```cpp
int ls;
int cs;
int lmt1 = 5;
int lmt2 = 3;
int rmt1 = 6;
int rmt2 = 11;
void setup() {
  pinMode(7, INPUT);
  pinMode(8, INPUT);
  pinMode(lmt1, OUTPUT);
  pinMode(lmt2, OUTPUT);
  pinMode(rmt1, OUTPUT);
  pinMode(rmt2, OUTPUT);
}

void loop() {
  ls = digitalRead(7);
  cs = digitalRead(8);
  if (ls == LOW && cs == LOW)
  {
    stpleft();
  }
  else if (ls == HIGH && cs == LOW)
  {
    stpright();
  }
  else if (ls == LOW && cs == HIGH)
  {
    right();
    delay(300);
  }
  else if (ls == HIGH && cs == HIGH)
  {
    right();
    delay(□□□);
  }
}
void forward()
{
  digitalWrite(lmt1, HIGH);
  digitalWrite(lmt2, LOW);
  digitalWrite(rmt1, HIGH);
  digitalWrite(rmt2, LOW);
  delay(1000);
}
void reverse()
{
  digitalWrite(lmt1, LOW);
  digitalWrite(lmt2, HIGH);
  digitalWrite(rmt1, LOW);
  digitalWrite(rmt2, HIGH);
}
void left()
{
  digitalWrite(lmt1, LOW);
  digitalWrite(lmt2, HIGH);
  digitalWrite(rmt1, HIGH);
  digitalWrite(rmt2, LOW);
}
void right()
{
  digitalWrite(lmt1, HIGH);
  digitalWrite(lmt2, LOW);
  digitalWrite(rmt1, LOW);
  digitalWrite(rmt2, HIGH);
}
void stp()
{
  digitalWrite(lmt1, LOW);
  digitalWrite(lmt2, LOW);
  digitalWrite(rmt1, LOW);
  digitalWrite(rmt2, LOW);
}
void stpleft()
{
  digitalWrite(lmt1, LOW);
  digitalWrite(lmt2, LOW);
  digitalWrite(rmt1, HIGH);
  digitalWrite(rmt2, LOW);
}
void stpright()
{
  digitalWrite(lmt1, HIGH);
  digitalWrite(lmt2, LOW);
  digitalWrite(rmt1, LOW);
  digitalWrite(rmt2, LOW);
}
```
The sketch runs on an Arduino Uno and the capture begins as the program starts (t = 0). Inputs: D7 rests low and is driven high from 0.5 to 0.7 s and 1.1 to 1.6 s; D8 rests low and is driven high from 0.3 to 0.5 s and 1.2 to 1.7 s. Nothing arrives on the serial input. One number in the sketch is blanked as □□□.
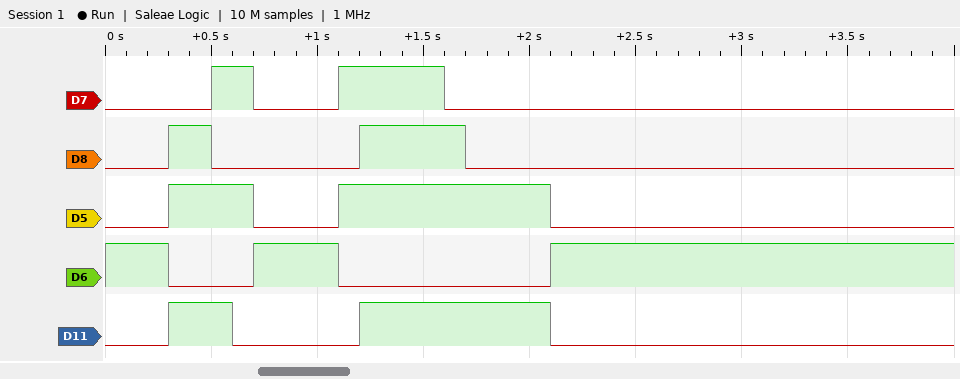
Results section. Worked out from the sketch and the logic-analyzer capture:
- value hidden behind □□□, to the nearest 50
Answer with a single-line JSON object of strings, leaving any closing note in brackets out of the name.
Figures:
{"value hidden behind □□□, to the nearest 50": "900"}
